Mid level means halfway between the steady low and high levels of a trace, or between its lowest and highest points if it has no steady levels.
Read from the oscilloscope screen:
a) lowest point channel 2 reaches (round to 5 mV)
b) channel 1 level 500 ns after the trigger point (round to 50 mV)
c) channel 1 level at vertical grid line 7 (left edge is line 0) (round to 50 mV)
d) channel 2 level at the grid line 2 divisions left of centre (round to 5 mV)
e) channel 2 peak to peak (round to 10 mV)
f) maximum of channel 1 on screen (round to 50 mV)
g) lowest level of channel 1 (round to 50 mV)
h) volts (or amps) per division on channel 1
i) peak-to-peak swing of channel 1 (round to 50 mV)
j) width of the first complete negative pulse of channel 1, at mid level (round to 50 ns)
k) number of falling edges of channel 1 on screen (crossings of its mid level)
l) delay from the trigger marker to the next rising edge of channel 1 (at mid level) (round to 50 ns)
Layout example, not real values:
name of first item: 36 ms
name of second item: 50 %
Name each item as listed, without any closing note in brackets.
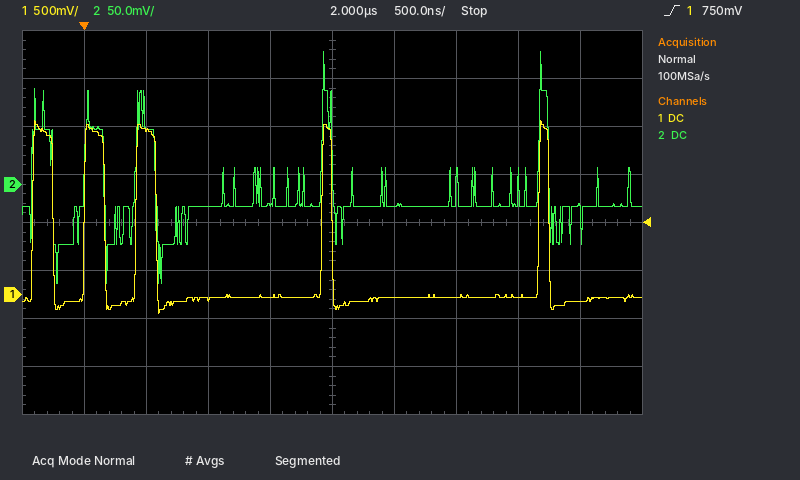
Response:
lowest point channel 2 reaches: -105 mV
channel 1 level 500 ns after the trigger point: 1.70 V
channel 1 level at vertical grid line 7 (left edge is line 0): -50 mV
channel 2 level at the grid line 2 divisions left of centre: -25 mV
channel 2 peak to peak: 240 mV
maximum of channel 1 on screen: 1.80 V
lowest level of channel 1: -200 mV
volts (or amps) per division on channel 1: 500 mV
peak-to-peak swing of channel 1: 2.00 V
width of the first complete negative pulse of channel 1, at mid level: 250 ns
number of falling edges of channel 1 on screen: 5
delay from the trigger marker to the next rising edge of channel 1 (at mid level): 400 ns
